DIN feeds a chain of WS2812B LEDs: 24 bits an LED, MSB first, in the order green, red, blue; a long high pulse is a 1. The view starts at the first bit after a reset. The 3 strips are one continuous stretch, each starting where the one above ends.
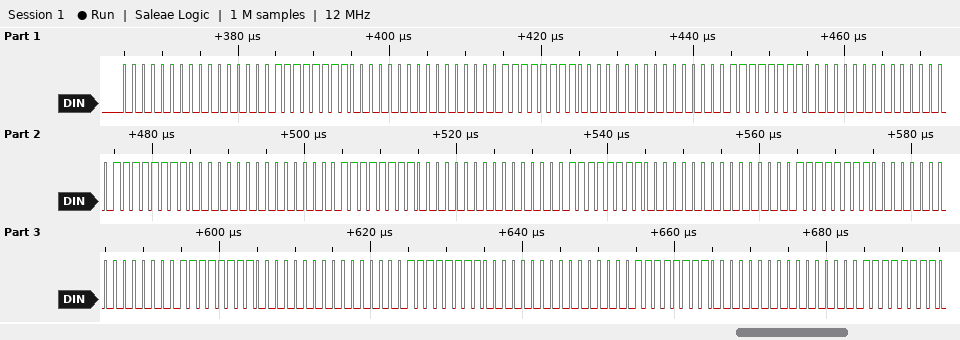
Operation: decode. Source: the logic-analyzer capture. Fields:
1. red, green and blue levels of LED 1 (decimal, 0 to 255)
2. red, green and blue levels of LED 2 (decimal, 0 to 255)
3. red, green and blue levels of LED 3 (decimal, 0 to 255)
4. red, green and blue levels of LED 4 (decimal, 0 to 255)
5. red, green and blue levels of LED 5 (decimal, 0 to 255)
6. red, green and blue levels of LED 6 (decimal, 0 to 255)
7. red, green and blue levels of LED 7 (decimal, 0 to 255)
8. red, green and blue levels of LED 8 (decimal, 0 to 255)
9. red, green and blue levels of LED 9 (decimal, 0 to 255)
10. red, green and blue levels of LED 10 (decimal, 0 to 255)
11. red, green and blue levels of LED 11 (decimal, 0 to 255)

0, 0, 255
0, 0, 255
0, 0, 255
0, 0, 255
0, 0, 255
0, 0, 255
0, 0, 255
0, 0, 255
0, 0, 255
0, 0, 255
0, 0, 255
